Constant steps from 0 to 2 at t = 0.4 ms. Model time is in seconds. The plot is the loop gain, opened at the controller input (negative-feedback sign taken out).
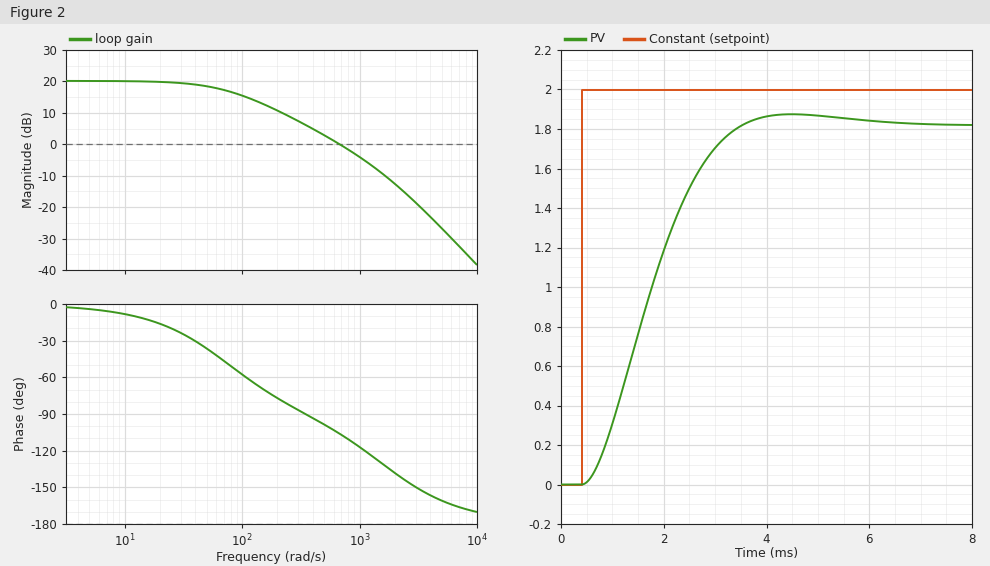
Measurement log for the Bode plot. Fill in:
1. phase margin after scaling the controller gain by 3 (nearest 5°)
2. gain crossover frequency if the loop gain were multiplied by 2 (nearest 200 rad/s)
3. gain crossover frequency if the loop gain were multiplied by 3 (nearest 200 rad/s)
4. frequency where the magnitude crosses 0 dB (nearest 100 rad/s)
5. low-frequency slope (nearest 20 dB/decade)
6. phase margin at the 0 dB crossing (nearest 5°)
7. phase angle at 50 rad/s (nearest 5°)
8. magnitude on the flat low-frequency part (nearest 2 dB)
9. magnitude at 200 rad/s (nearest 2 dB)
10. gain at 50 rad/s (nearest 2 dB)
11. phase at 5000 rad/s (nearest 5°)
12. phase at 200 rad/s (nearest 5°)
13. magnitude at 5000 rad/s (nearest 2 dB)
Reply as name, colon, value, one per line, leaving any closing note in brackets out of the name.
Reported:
phase margin after scaling the controller gain by 3: 50°
gain crossover frequency if the loop gain were multiplied by 2: 1200 rad/s
gain crossover frequency if the loop gain were multiplied by 3: 1600 rad/s
frequency where the magnitude crosses 0 dB: 700 rad/s
low-frequency slope: 0 dB/decade
phase margin at the 0 dB crossing: 75°
phase angle at 50 rad/s: -35°
magnitude on the flat low-frequency part: 20 dB
magnitude at 200 rad/s: 10 dB
gain at 50 rad/s: 18 dB
phase at 5000 rad/s: -160°
phase at 200 rad/s: -75°
magnitude at 5000 rad/s: -26 dB
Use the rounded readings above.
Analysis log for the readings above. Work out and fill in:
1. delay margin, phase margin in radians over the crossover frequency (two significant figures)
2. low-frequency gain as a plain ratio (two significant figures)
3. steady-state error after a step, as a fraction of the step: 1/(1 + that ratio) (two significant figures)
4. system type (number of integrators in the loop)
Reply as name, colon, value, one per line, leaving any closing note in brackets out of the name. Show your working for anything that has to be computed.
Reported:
delay margin, phase margin in radians over the crossover frequency: 75 × π / 180 / 700 = 0.0019 s
low-frequency gain as a plain ratio: 10^(20 / 20) = 10
steady-state error after a step, as a fraction of the step: 1/(1 + that ratio): 1 / (1 + 10) = 0.091
system type: 0
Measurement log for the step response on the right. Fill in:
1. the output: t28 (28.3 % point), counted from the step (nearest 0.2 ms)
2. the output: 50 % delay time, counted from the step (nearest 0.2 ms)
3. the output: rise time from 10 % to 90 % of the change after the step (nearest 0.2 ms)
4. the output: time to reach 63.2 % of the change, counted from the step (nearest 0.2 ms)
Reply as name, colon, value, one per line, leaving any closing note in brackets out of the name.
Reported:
the output: t28 (28.3 % point), counted from the step: 0.8 ms
the output: 50 % delay time, counted from the step: 1.2 ms
the output: rise time from 10 % to 90 % of the change after the step: 2.0 ms
the output: time to reach 63.2 % of the change, counted from the step: 1.6 ms
